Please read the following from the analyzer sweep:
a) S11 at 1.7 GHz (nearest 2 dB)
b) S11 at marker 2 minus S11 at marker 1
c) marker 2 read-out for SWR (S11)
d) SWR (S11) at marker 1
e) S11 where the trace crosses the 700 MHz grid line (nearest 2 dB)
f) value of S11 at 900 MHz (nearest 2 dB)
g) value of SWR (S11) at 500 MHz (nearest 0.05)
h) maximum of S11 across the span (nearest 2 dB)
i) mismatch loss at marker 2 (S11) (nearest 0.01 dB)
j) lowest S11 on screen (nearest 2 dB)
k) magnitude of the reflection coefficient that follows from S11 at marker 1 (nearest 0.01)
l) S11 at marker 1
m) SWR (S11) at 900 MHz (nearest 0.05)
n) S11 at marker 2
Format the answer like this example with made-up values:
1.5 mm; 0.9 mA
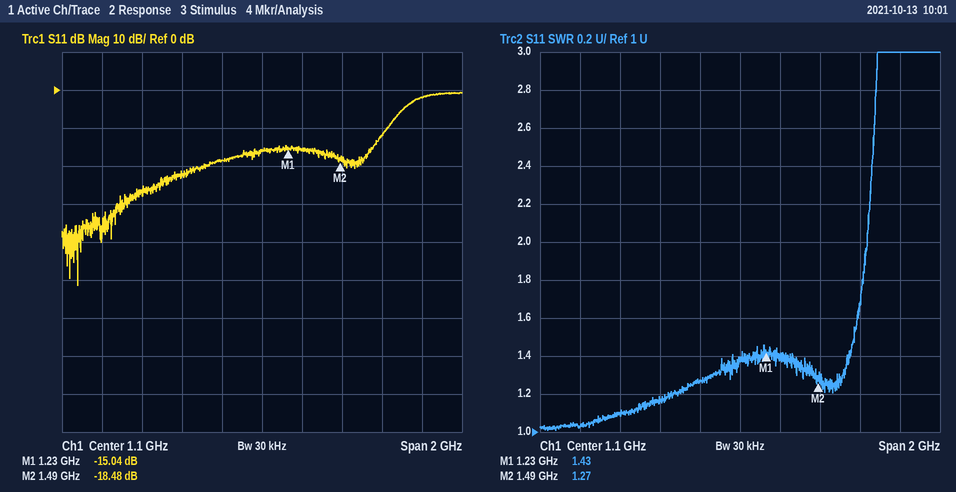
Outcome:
-12 dB; -3.44 dB; 1.27; 1.43; -22 dB; -18 dB; 1.10; 0 dB; 0.06 dB; -52 dB; 0.18; -15.04 dB; 1.25; -18.48 dB
